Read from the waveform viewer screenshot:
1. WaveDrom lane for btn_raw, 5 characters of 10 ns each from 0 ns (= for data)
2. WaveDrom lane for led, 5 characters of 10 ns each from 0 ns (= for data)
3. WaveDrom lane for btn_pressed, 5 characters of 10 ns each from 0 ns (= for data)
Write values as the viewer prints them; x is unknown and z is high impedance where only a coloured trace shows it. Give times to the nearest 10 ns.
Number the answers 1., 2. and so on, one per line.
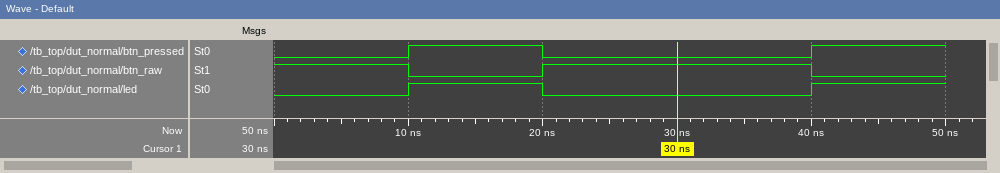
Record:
1. {name: 'btn_raw', wave: '101.0'}
2. {name: 'led', wave: '010.1'}
3. {name: 'btn_pressed', wave: '010.1'}
